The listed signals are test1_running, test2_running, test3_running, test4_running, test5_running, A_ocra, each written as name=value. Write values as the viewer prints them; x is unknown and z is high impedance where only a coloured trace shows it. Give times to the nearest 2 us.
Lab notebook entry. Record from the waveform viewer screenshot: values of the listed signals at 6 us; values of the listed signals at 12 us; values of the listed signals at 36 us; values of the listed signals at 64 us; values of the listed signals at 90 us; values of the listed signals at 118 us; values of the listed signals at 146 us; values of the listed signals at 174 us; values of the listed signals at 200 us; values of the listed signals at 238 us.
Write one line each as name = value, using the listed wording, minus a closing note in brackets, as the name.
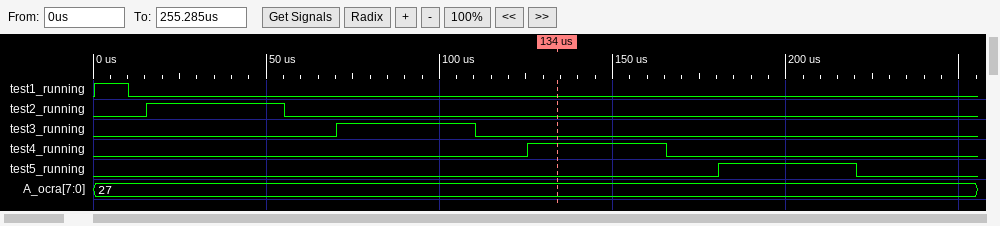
values of the listed signals at 6 us = test1_running=1, test2_running=0, test3_running=0, test4_running=0, test5_running=0, A_ocra=27
values of the listed signals at 12 us = test1_running=0, test2_running=0, test3_running=0, test4_running=0, test5_running=0, A_ocra=27
values of the listed signals at 36 us = test1_running=0, test2_running=1, test3_running=0, test4_running=0, test5_running=0, A_ocra=27
values of the listed signals at 64 us = test1_running=0, test2_running=0, test3_running=0, test4_running=0, test5_running=0, A_ocra=27
values of the listed signals at 90 us = test1_running=0, test2_running=0, test3_running=1, test4_running=0, test5_running=0, A_ocra=27
values of the listed signals at 118 us = test1_running=0, test2_running=0, test3_running=0, test4_running=0, test5_running=0, A_ocra=27
values of the listed signals at 146 us = test1_running=0, test2_running=0, test3_running=0, test4_running=1, test5_running=0, A_ocra=27
values of the listed signals at 174 us = test1_running=0, test2_running=0, test3_running=0, test4_running=0, test5_running=0, A_ocra=27
values of the listed signals at 200 us = test1_running=0, test2_running=0, test3_running=0, test4_running=0, test5_running=1, A_ocra=27
values of the listed signals at 238 us = test1_running=0, test2_running=0, test3_running=0, test4_running=0, test5_running=0, A_ocra=27
